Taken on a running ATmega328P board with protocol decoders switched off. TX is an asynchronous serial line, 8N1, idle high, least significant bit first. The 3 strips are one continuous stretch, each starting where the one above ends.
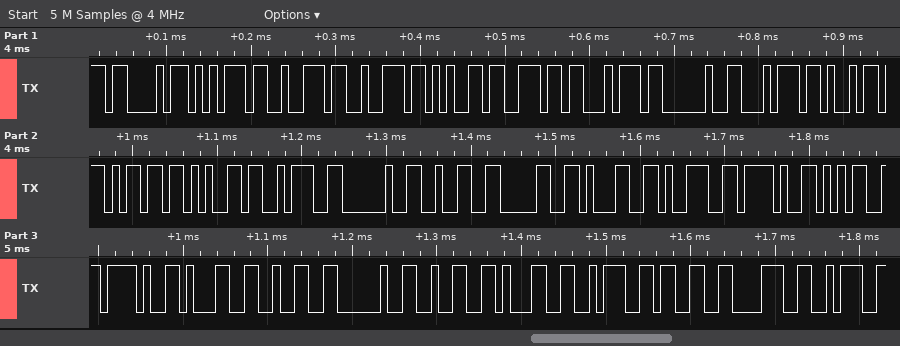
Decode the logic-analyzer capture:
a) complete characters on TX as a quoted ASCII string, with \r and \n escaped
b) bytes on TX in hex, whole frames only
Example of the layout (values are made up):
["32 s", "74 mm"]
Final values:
["\"Current time: 2019/5/12 21:38:\"", "43 75 72 72 65 6E 74 20 74 69 6D 65 3A 20 32 30 31 39 2F 35 2F 31 32 20 32 31 3A 33 38 3A"]
